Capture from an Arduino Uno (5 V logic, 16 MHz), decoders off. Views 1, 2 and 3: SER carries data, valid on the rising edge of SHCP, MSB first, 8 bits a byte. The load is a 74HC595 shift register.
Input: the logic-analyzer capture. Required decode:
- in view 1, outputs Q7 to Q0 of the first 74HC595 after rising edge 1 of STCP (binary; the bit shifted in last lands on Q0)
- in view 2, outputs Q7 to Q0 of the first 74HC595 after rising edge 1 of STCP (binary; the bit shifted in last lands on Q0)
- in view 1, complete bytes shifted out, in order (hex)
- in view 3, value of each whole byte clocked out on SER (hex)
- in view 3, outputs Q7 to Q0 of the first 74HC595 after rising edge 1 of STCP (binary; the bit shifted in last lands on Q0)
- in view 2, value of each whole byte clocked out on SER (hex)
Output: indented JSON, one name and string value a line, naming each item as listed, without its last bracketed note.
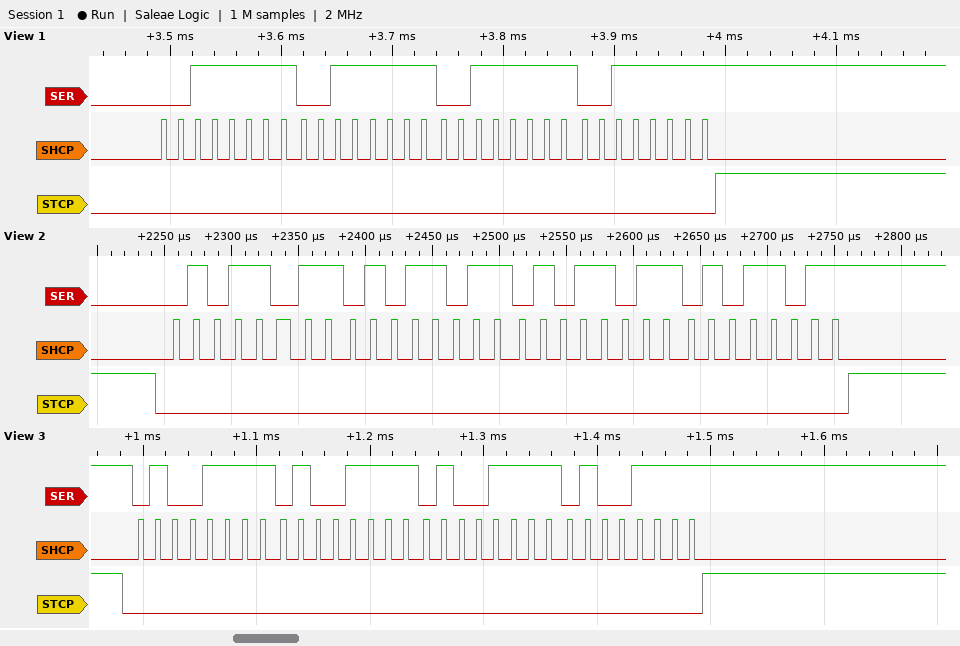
{
  "in view 1, outputs Q7 to Q0 of the first 74HC595 after rising edge 1 of STCP": "00111111",
  "in view 2, outputs Q7 to Q0 of the first 74HC595 after rising edge 1 of STCP": "01011011",
  "in view 1, complete bytes shifted out, in order": "0x3F 0x3F 0x3F 0x3F",
  "in view 3, value of each whole byte clocked out on SER": "4F 4F 4F 4F",
  "in view 3, outputs Q7 to Q0 of the first 74HC595 after rising edge 1 of STCP": "01001111",
  "in view 2, value of each whole byte clocked out on SER": "0x5B 0x5B 0x5B 0x5B"
}
